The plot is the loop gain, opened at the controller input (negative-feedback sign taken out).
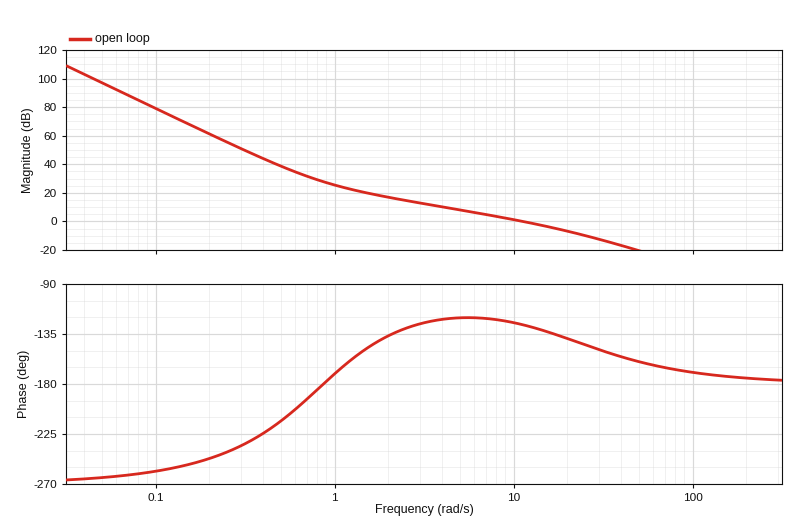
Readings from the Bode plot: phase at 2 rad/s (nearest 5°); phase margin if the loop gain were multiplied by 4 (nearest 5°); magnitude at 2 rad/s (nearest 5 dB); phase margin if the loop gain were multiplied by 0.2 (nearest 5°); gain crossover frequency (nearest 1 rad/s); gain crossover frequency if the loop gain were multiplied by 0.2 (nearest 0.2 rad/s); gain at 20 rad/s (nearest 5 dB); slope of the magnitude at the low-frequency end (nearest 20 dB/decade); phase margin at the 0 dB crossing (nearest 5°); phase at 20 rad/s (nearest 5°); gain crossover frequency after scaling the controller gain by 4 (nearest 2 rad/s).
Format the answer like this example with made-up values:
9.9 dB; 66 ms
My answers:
-135°; 30°; 15 dB; 50°; 11 rad/s; 2.6 rad/s; -5 dB; -60 dB/decade; 55°; -140°; 30 rad/s
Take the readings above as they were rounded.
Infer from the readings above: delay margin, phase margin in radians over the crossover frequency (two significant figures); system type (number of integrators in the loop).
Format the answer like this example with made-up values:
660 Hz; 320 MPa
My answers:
0.087 s; 3
